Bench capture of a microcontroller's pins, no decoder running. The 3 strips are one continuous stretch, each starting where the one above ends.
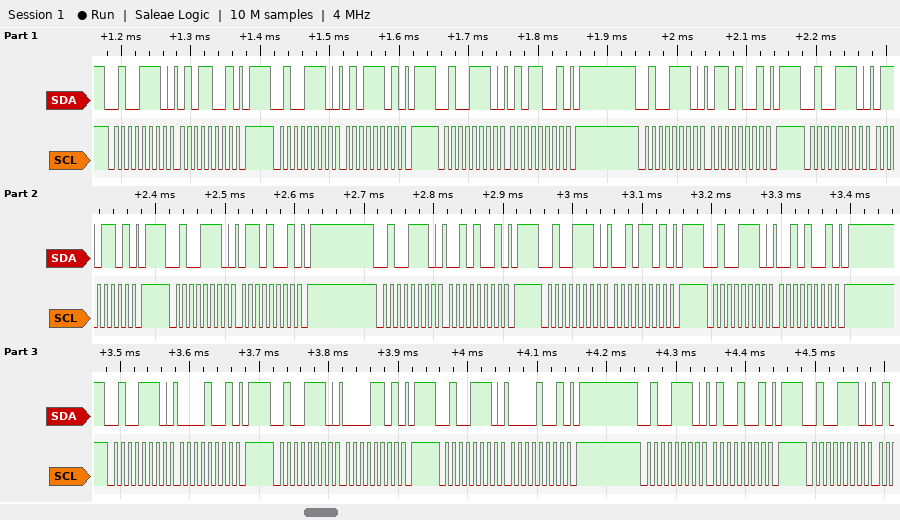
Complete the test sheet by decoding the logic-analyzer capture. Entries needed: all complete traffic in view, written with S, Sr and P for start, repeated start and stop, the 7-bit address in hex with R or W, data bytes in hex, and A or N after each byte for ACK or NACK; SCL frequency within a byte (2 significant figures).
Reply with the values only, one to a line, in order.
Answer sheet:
S 27W A 59 A P S 27W A 5D A P S 27W A 59 A P S 27W A 69 A P S 27W A 6D A P S 27W A 69 A P S 27W A 29 A P S 27W A 2D A P S 27W A 29 A P S 27W A 09 A P S 27W A 0D A P S 27W A 09 A P S 27W A 49 A P S 27W A
100 kHz
